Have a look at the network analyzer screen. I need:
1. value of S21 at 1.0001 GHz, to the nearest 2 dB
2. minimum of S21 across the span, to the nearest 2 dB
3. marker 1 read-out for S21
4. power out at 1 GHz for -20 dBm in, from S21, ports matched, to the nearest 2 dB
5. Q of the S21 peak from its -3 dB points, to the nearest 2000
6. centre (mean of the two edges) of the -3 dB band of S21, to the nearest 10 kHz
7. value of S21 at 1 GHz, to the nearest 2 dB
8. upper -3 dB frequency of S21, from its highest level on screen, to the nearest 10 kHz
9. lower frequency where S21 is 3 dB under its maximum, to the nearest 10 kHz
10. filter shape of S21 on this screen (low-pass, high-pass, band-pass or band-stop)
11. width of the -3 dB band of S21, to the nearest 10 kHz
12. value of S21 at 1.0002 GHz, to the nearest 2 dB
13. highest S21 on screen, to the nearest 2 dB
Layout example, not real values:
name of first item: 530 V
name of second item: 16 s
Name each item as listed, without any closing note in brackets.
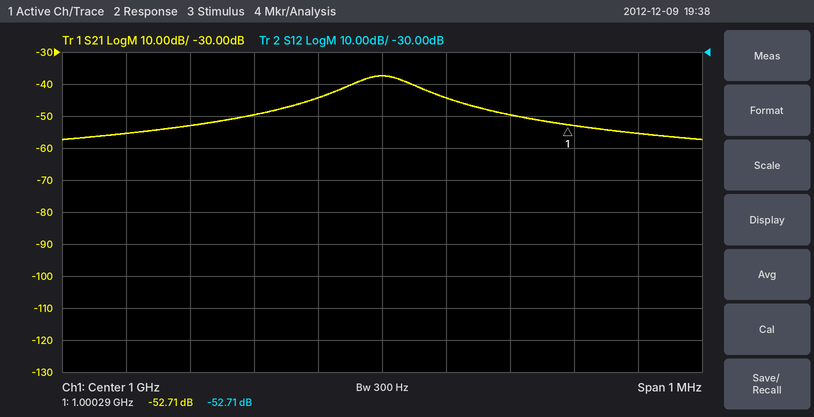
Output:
value of S21 at 1.0001 GHz, to the nearest 2 dB: -44 dB
minimum of S21 across the span, to the nearest 2 dB: -58 dB
marker 1 read-out for S21: -52.71 dB
power out at 1 GHz for -20 dBm in, from S21, ports matched, to the nearest 2 dB: -58 dBm
Q of the S21 peak from its -3 dB points, to the nearest 2000: 10000
centre (mean of the two edges) of the -3 dB band of S21, to the nearest 10 kHz: 1.00000 GHz
value of S21 at 1 GHz, to the nearest 2 dB: -38 dB
upper -3 dB frequency of S21, from its highest level on screen, to the nearest 10 kHz: 1.00005 GHz
lower frequency where S21 is 3 dB under its maximum, to the nearest 10 kHz: 999.95 MHz
filter shape of S21 on this screen: band-pass
width of the -3 dB band of S21, to the nearest 10 kHz: 100 kHz
value of S21 at 1.0002 GHz, to the nearest 2 dB: -50 dB
highest S21 on screen, to the nearest 2 dB: -38 dB
